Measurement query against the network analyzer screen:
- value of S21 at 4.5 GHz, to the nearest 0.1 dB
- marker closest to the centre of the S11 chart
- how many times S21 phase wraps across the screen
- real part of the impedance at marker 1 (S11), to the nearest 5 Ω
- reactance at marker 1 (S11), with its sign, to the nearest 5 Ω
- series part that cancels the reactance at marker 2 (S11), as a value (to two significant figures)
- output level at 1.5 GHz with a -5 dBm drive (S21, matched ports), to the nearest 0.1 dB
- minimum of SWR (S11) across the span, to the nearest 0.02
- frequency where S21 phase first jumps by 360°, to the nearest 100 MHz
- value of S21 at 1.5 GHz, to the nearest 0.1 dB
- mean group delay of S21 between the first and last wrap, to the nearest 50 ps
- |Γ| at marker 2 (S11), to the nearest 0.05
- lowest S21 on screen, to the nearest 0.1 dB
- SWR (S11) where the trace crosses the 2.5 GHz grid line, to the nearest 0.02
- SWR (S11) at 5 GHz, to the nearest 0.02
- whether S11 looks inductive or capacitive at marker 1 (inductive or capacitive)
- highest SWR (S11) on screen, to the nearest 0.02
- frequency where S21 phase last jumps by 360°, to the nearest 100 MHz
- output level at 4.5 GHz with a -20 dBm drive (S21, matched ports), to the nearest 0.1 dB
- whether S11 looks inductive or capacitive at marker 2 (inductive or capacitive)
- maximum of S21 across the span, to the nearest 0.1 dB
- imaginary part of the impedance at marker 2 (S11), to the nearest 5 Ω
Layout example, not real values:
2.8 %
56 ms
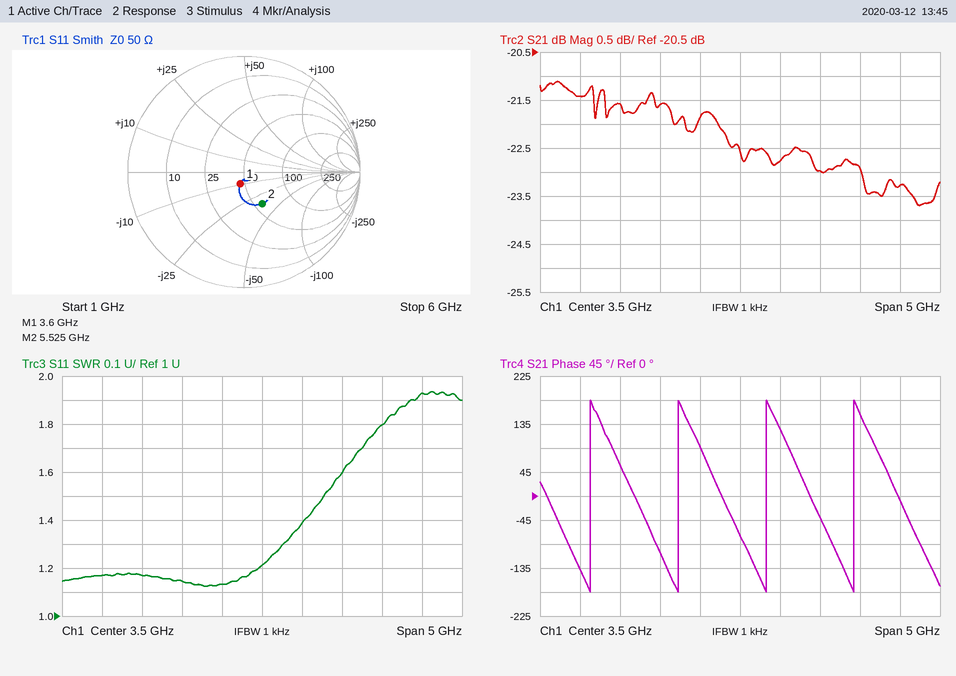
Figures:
-23.0 dB
marker 1
4
45 Ω
-10 Ω
1.0 nH
-26.4 dBm
1.12
1.6 GHz
-21.4 dB
900 ps
0.30
-23.7 dB
1.14
1.80
capacitive
1.94
4.9 GHz
-43.0 dBm
capacitive
-21.1 dB
-35 Ω
